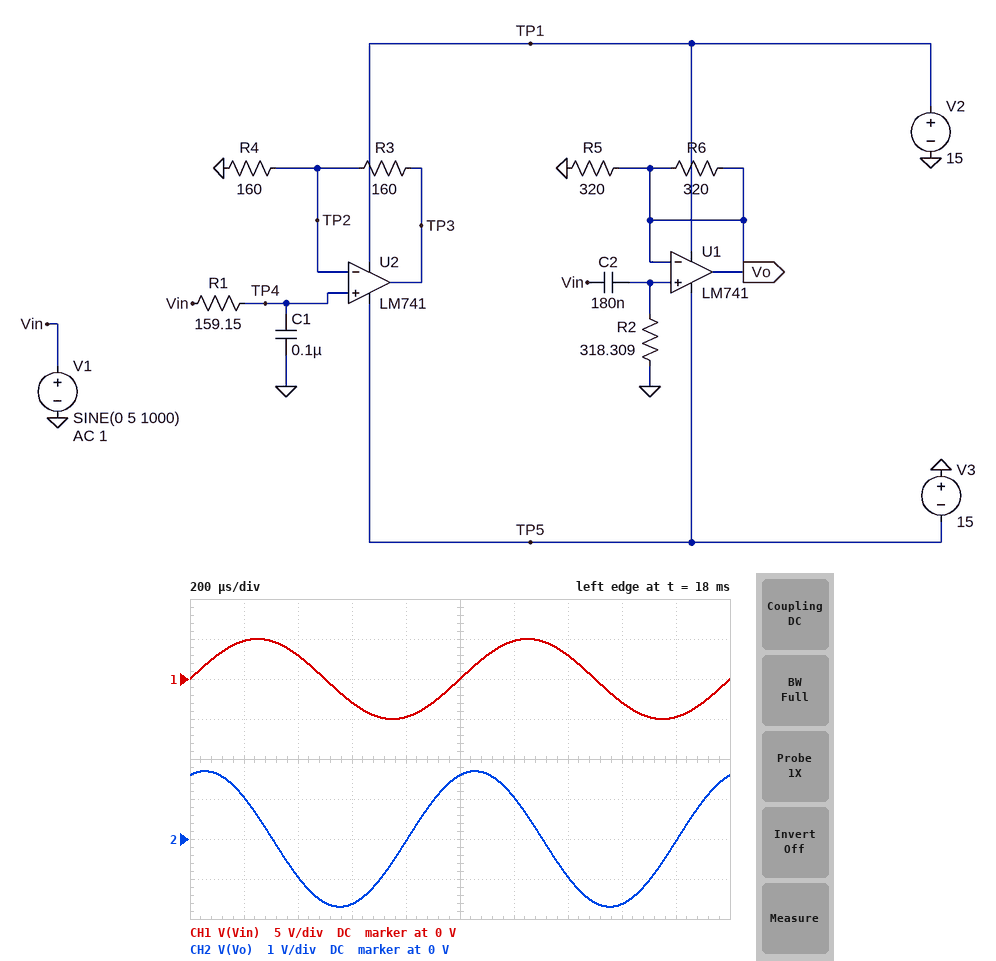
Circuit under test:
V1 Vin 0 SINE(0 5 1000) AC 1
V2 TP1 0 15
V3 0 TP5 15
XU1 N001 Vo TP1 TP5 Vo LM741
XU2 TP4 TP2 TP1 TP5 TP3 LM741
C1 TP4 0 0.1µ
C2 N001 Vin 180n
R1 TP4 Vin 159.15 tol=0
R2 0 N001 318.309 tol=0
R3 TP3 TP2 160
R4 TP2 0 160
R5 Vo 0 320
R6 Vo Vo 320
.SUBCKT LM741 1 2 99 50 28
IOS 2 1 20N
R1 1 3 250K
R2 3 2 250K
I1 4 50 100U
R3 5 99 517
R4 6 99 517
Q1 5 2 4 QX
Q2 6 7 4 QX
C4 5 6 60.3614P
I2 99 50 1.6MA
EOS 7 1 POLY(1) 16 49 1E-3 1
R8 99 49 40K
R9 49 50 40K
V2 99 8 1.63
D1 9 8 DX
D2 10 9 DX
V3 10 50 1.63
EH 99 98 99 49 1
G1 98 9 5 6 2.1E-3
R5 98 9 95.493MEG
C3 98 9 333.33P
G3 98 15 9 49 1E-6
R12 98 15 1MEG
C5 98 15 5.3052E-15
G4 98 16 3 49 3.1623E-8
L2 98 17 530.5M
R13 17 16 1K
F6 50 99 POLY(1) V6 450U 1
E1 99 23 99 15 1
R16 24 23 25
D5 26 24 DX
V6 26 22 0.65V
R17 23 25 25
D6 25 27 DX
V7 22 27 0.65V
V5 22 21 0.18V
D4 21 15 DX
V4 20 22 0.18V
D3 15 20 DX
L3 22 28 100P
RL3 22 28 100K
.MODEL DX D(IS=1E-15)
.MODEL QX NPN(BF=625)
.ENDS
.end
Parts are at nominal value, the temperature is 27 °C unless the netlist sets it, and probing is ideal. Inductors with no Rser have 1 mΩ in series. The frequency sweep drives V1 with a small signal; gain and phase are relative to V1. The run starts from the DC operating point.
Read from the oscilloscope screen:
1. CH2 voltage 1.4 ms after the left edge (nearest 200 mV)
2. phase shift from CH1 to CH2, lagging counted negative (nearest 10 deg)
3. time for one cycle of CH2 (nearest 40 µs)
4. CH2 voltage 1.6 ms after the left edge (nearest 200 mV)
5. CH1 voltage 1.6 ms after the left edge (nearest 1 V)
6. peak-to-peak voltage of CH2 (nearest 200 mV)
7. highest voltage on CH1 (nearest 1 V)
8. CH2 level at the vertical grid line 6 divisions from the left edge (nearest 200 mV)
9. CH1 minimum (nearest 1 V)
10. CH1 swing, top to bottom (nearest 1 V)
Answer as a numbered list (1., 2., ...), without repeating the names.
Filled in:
1. -1.0 V
2. 70 deg
3. 1.00 ms
4. -1.6 V
5. -3 V
6. 3.4 V
7. 5 V
8. 1.0 V
9. -5 V
10. 10 V
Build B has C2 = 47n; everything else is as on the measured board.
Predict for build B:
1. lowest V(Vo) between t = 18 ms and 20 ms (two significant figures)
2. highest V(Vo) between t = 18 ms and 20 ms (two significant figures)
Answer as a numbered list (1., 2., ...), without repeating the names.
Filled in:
1. -470 mV
2. 470 mV
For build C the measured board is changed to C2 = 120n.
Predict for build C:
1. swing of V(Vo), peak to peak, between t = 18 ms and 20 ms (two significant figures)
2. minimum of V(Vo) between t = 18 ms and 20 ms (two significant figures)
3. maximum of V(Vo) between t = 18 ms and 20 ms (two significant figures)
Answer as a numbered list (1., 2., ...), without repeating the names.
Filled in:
1. 2.3 V
2. -1.2 V
3. 1.2 V
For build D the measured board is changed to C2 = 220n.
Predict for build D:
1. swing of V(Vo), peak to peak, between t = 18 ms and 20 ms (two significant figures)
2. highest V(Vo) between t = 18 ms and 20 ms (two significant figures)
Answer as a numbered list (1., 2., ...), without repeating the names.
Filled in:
1. 4.0 V
2. 2.0 V
